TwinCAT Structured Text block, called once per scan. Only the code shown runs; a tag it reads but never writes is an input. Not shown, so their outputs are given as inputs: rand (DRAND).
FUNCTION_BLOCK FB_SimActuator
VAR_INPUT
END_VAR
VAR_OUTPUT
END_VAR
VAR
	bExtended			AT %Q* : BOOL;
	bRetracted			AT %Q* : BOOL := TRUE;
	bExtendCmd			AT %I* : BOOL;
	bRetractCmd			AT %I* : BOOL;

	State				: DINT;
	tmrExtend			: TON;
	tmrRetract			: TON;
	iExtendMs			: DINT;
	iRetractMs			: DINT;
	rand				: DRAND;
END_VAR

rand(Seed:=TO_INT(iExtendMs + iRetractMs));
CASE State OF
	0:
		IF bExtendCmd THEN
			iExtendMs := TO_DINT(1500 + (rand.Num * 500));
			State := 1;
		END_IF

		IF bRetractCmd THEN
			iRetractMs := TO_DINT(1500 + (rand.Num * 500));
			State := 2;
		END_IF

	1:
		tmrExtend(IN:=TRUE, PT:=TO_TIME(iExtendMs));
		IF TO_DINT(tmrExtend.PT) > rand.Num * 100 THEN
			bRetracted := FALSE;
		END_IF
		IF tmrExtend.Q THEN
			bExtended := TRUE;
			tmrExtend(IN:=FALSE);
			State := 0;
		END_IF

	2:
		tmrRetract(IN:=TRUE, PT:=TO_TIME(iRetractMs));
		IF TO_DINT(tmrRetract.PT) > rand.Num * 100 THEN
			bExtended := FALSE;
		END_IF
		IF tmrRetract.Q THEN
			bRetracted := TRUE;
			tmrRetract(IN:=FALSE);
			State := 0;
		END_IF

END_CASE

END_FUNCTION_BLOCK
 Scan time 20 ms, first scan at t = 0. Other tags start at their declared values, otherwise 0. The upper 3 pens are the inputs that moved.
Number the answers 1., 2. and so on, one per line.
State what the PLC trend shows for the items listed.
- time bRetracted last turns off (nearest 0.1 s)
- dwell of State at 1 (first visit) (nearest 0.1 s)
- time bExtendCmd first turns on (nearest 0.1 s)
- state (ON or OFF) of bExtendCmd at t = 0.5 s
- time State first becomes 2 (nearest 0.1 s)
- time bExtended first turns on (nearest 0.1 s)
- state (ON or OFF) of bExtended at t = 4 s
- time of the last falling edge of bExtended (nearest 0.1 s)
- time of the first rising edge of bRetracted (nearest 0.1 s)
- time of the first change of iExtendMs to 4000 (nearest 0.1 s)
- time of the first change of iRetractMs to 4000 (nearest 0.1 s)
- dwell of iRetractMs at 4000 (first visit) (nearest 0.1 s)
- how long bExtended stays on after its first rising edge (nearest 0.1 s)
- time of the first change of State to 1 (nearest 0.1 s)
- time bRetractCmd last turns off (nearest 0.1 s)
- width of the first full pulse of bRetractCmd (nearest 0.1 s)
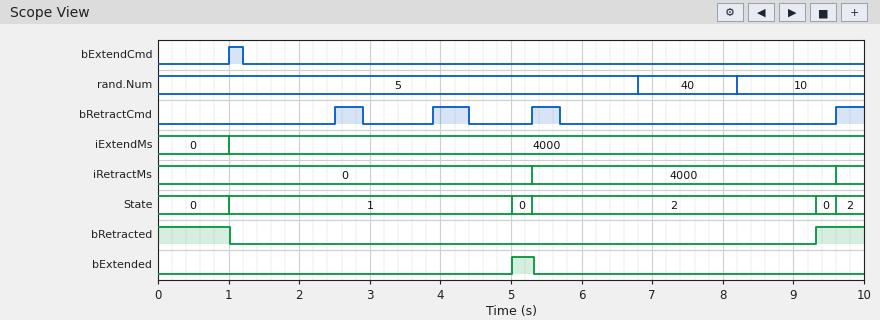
1. 1.0 s
2. 4.0 s
3. 1.0 s
4. OFF
5. 5.3 s
6. 5.0 s
7. OFF
8. 5.3 s
9. 9.3 s
10. 1.0 s
11. 5.3 s
12. 4.3 s
13. 0.3 s
14. 1.0 s
15. 5.7 s
16. 0.4 s
